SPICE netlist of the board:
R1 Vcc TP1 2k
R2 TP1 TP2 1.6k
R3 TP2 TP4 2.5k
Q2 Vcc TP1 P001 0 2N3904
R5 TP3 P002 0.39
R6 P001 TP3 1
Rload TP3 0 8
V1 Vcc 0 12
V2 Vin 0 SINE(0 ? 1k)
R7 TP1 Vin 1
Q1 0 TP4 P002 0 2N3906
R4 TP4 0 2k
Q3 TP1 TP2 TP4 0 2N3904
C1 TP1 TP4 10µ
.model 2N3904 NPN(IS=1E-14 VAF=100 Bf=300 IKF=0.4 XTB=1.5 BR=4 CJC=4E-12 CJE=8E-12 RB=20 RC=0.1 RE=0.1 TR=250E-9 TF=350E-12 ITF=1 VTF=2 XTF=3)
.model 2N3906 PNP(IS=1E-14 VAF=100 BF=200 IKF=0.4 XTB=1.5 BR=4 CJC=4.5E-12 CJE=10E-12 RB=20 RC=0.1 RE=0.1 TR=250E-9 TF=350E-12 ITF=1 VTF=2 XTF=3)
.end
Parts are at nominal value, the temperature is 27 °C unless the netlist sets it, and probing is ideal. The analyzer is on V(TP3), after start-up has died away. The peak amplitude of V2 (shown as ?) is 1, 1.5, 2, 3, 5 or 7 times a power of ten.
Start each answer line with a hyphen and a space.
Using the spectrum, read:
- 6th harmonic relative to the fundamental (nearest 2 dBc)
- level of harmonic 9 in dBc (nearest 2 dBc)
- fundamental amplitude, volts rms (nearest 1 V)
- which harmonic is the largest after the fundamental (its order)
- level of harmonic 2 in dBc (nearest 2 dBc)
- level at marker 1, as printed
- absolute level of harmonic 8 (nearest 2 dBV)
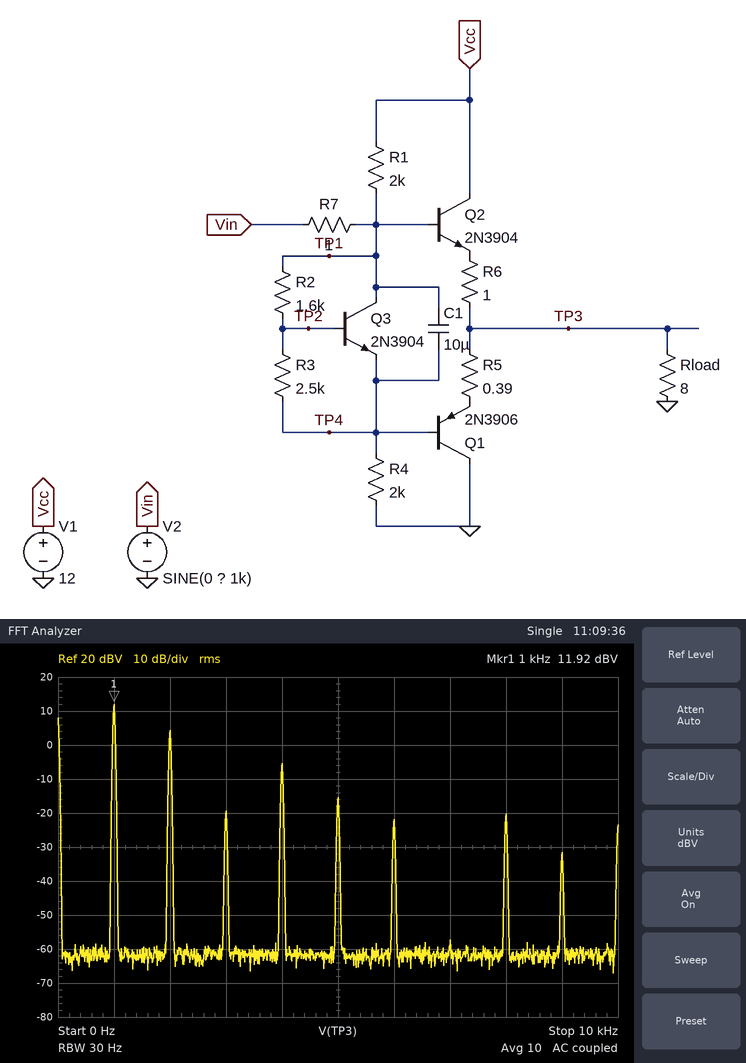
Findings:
- -34 dBc
- -44 dBc
- 4 V
- 2
- -8 dBc
- 11.92 dBV
- -20 dBV
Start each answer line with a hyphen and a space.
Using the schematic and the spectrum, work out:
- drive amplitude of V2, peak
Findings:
- 15 V
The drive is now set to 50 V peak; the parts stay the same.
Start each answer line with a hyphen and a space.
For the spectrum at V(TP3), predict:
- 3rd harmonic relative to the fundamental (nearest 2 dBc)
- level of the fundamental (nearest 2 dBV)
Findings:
- -10 dBc
- 14 dBV
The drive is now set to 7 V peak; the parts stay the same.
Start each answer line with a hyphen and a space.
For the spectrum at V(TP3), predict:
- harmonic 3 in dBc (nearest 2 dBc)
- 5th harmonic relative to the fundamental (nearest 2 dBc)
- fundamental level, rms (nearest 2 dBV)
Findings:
- -26 dBc
- -30 dBc
- 6 dBV
